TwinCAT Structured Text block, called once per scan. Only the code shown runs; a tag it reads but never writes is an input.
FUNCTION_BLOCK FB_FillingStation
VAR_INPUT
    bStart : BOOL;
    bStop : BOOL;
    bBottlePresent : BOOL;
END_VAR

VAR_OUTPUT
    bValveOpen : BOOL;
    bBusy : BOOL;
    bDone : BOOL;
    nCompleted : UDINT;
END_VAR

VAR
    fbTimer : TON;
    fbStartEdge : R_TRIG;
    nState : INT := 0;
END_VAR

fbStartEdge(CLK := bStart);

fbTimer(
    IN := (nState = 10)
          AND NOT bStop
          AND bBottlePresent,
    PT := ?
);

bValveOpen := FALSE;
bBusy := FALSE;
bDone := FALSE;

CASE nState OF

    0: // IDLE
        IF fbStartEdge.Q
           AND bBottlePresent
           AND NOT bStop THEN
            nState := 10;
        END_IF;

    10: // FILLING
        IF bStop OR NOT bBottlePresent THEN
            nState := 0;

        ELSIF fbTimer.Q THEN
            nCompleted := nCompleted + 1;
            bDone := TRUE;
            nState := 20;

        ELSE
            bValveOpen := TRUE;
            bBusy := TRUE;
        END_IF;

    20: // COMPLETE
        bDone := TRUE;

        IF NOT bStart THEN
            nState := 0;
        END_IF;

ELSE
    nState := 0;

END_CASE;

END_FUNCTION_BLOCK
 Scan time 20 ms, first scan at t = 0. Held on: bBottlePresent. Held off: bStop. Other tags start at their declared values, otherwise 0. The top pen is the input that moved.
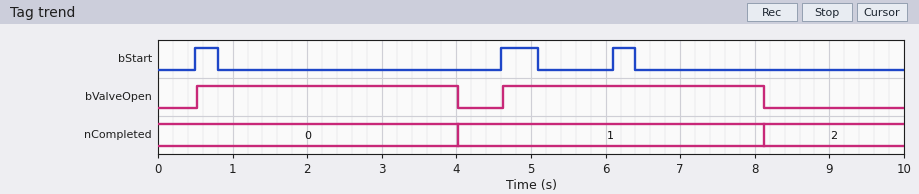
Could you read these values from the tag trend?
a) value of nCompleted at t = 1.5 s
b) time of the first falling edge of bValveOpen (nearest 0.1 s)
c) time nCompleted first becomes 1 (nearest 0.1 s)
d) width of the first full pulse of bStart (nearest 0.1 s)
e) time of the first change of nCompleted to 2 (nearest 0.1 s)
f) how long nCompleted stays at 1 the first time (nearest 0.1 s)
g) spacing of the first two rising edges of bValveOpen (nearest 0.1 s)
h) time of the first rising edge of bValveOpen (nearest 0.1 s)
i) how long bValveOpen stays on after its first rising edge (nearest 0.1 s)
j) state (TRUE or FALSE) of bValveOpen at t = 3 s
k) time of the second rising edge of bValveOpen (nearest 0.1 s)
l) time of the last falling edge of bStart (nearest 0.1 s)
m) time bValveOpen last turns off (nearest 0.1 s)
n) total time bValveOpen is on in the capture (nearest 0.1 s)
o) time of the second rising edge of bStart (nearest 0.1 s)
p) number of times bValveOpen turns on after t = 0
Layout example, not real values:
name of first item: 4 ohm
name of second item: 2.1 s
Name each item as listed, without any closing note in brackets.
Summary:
value of nCompleted at t = 1.5 s: 0
time of the first falling edge of bValveOpen: 4.0 s
time nCompleted first becomes 1: 4.0 s
width of the first full pulse of bStart: 0.3 s
time of the first change of nCompleted to 2: 8.1 s
how long nCompleted stays at 1 the first time: 4.1 s
spacing of the first two rising edges of bValveOpen: 4.1 s
time of the first rising edge of bValveOpen: 0.5 s
how long bValveOpen stays on after its first rising edge: 3.5 s
state (TRUE or FALSE) of bValveOpen at t = 3 s: TRUE
time of the second rising edge of bValveOpen: 4.6 s
time of the last falling edge of bStart: 6.4 s
time bValveOpen last turns off: 8.1 s
total time bValveOpen is on in the capture: 7.0 s
time of the second rising edge of bStart: 4.6 s
number of times bValveOpen turns on after t = 0: 2
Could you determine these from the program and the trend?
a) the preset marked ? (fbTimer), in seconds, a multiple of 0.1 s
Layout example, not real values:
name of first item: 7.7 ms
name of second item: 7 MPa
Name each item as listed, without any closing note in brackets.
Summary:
the preset marked ? (fbTimer), in seconds, a multiple of 0.1 s: 3.5 s
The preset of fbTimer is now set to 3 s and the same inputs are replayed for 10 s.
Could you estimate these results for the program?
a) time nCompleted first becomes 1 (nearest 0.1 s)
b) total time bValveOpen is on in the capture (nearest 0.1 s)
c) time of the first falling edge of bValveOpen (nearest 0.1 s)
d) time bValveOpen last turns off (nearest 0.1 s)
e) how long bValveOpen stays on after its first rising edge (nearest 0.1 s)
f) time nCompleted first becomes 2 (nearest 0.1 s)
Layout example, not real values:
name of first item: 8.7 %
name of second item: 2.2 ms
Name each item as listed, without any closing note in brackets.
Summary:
time nCompleted first becomes 1: 3.5 s
total time bValveOpen is on in the capture: 6.0 s
time of the first falling edge of bValveOpen: 3.5 s
time bValveOpen last turns off: 7.6 s
how long bValveOpen stays on after its first rising edge: 3.0 s
time nCompleted first becomes 2: 7.6 s
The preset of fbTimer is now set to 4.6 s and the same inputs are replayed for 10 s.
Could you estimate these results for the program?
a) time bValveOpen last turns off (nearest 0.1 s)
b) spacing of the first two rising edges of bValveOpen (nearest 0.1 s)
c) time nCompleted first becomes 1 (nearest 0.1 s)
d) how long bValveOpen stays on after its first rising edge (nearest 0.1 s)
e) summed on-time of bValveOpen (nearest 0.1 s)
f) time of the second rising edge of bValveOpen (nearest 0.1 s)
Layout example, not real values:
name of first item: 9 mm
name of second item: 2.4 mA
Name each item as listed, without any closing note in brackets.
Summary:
time bValveOpen last turns off: 5.1 s
spacing of the first two rising edges of bValveOpen: 5.6 s
time nCompleted first becomes 1: 5.1 s
how long bValveOpen stays on after its first rising edge: 4.6 s
summed on-time of bValveOpen: 8.5 s
time of the second rising edge of bValveOpen: 6.1 s
